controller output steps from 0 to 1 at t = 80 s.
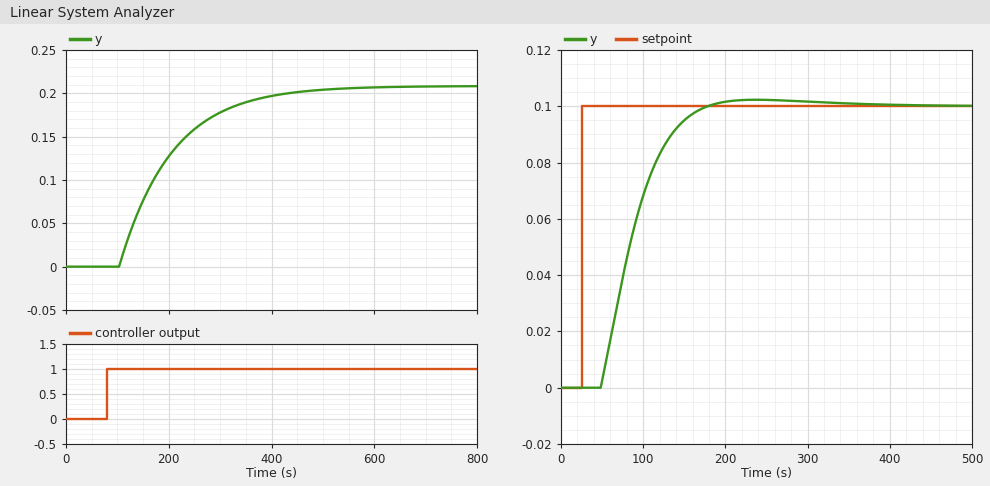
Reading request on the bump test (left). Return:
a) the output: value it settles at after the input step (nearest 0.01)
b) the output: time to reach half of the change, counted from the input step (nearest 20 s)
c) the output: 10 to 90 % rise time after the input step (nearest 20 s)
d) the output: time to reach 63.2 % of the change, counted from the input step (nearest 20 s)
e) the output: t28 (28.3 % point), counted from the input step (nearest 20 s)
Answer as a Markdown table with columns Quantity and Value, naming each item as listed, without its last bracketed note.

| Quantity | Value |
|---|---|
| the output: value it settles at after the input step | 0.21 |
| the output: time to reach half of the change, counted from the input step | 100 s |
| the output: 10 to 90 % rise time after the input step | 220 s |
| the output: time to reach 63.2 % of the change, counted from the input step | 120 s |
| the output: t28 (28.3 % point), counted from the input step | 60 s |
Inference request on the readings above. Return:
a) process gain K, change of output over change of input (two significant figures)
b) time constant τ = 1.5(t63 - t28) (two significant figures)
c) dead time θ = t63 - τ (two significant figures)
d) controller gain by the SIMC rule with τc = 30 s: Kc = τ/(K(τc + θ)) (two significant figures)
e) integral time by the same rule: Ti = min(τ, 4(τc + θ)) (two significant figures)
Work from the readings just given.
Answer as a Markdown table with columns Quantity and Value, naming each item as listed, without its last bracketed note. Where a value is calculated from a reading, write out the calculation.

| Quantity | Value |
|---|---|
| process gain K, change of output over change of input | (0.21 - 0) / 1 = 0.21 |
| time constant τ = 1.5(t63 - t28) | 1.5 × (120 - 60) = 90 s |
| dead time θ = t63 - τ | 120 - 90 = 30 s |
| controller gain by the SIMC rule with τc = 30 s: Kc = τ/(K(τc + θ)) | 90 / (0.21 × (30 + 30)) = 7.1 |
| integral time by the same rule: Ti = min(τ, 4(τc + θ)) | min(90, 4 × (30 + 30)) = 90 s |
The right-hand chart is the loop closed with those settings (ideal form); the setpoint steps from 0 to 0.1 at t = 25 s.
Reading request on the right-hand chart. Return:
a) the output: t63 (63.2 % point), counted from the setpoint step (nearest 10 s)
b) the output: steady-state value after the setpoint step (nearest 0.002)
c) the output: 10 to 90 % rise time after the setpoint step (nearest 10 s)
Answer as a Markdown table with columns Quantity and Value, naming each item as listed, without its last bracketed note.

| Quantity | Value |
|---|---|
| the output: t63 (63.2 % point), counted from the setpoint step | 70 s |
| the output: steady-state value after the setpoint step | 0.100 |
| the output: 10 to 90 % rise time after the setpoint step | 80 s |
